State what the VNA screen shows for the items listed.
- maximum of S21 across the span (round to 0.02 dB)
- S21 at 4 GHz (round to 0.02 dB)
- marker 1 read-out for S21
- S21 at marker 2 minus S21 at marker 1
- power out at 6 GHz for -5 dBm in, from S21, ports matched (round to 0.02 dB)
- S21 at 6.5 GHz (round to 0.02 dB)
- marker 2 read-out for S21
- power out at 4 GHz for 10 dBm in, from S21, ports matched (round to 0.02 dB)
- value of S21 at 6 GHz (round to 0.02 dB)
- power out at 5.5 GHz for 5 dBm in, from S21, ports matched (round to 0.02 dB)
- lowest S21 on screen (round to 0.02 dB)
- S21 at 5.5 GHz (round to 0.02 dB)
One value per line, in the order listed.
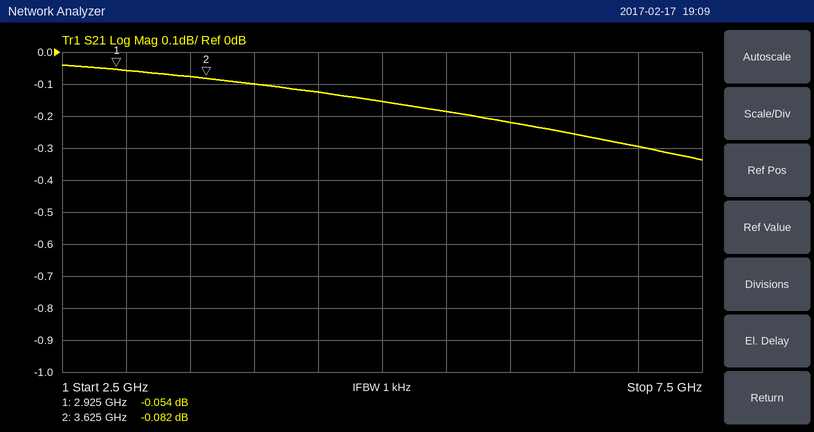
-0.04 dB
-0.10 dB
-0.054 dB
-0.028 dB
-5.22 dBm
-0.26 dB
-0.082 dB
9.90 dBm
-0.22 dB
4.82 dBm
-0.34 dB
-0.18 dB
